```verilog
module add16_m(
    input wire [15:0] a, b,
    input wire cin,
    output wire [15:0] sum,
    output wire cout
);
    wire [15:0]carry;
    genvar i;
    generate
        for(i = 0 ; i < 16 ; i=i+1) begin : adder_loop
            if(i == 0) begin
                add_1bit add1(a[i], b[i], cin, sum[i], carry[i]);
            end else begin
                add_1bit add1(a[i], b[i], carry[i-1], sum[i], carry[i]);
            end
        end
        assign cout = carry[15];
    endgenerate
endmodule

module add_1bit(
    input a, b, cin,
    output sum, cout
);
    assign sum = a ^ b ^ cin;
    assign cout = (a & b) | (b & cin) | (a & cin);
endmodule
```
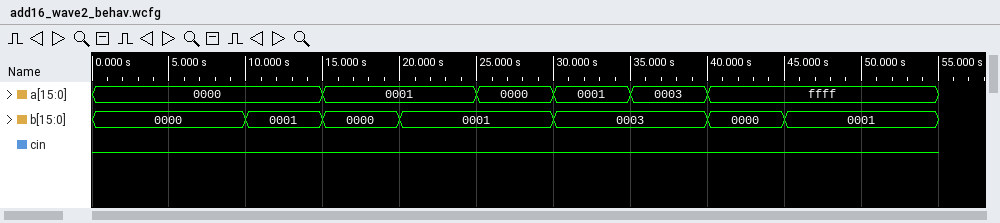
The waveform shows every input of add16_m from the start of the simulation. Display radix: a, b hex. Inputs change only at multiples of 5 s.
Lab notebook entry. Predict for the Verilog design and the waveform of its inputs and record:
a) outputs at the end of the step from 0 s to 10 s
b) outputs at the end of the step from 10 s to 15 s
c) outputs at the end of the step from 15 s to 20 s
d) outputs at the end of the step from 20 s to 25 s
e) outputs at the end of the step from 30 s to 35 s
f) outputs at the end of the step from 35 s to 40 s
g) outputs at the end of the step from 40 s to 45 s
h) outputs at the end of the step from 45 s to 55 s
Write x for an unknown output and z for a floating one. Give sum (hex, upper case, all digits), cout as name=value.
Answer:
sum=0000, cout=0
sum=0001, cout=0
sum=0001, cout=0
sum=0002, cout=0
sum=0004, cout=0
sum=0006, cout=0
sum=FFFF, cout=0
sum=0000, cout=1
